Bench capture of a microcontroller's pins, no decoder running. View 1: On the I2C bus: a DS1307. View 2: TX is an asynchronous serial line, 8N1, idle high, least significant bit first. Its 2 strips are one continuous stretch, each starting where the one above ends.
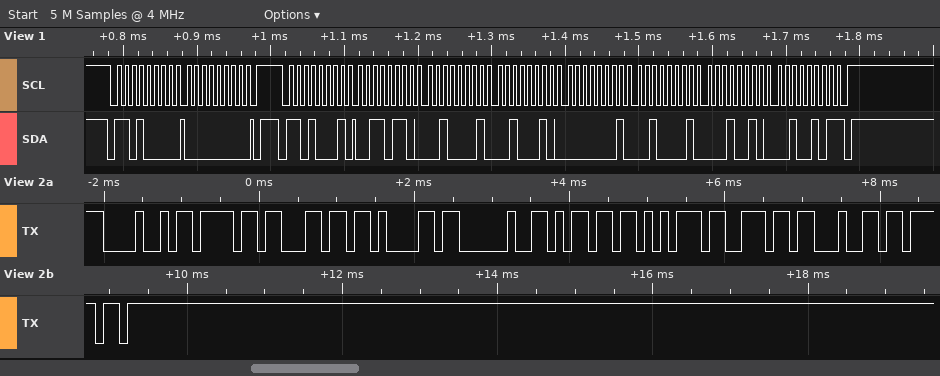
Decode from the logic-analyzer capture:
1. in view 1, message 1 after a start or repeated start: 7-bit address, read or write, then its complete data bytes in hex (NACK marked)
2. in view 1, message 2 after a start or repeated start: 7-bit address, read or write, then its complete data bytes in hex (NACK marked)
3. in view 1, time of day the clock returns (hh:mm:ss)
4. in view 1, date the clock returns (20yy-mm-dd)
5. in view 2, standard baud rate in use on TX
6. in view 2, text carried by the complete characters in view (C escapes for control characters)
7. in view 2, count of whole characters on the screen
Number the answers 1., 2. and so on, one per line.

1. 0x68 write: 00
2. 0x68 read: 36 21 22 01 21 12 25 NACK
3. 22:21:36
4. 2025-12-21
5. 9600 baud
6. "Hola mundo"
7. 10
